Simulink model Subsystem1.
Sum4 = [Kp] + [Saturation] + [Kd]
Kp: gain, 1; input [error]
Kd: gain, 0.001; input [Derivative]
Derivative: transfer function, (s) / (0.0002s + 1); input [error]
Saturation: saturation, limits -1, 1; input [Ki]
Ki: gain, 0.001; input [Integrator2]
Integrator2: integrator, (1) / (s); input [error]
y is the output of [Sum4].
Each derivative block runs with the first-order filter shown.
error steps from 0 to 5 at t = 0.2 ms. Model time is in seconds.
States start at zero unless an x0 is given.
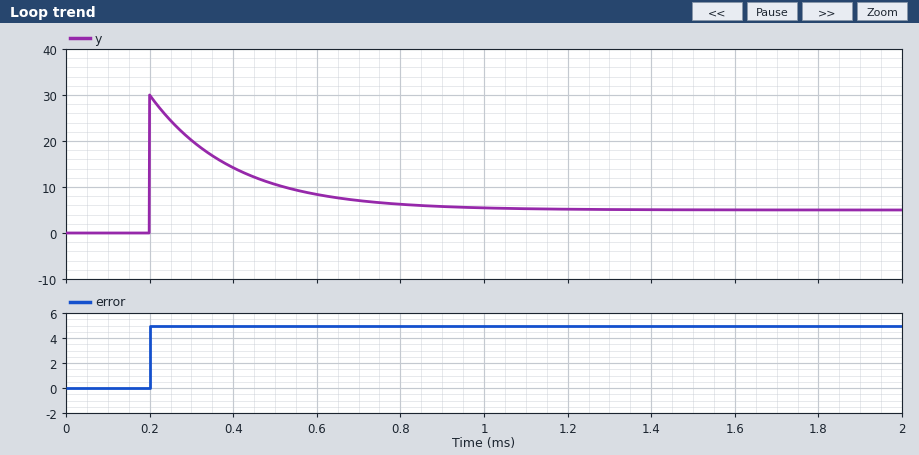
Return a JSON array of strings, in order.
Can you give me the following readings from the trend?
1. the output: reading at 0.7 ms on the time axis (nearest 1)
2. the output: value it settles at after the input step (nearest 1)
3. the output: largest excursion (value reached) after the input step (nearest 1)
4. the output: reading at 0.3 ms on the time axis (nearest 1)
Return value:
["7", "5", "30", "20"]
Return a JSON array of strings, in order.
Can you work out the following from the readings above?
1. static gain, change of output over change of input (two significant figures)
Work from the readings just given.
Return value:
["1.0"]
